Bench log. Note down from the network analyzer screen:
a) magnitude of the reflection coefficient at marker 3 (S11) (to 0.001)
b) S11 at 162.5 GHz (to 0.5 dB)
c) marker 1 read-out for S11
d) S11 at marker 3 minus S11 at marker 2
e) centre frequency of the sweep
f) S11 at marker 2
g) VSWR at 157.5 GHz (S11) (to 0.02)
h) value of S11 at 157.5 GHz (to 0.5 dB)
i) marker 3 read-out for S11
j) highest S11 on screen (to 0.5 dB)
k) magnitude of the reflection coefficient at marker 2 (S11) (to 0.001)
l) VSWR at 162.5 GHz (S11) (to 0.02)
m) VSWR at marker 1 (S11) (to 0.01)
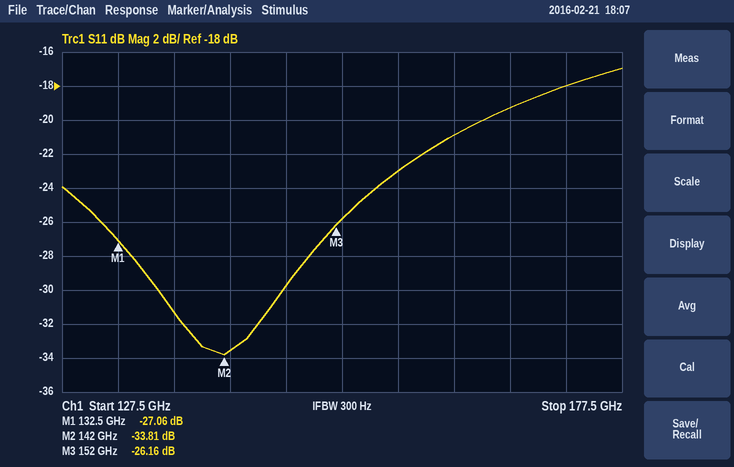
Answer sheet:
0.049
-21.0 dB
-27.06 dB
7.65 dB
152.5 GHz
-33.81 dB
1.16
-23.0 dB
-26.16 dB
-17.0 dB
0.020
1.20
1.09
